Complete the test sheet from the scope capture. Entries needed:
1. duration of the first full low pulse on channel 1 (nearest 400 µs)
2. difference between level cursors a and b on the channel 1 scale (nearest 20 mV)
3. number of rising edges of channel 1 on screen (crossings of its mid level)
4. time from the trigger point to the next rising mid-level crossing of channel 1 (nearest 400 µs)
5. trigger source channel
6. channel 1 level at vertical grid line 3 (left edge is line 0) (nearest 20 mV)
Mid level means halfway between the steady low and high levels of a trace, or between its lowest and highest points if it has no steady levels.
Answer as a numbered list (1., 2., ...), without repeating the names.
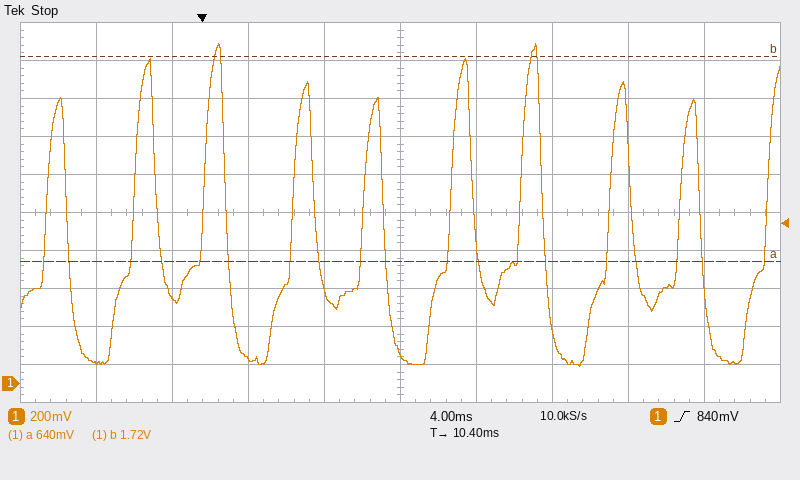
1. 3.6 ms
2. 1.08 V
3. 10
4. 4.8 ms
5. channel 1
6. 140 mV
